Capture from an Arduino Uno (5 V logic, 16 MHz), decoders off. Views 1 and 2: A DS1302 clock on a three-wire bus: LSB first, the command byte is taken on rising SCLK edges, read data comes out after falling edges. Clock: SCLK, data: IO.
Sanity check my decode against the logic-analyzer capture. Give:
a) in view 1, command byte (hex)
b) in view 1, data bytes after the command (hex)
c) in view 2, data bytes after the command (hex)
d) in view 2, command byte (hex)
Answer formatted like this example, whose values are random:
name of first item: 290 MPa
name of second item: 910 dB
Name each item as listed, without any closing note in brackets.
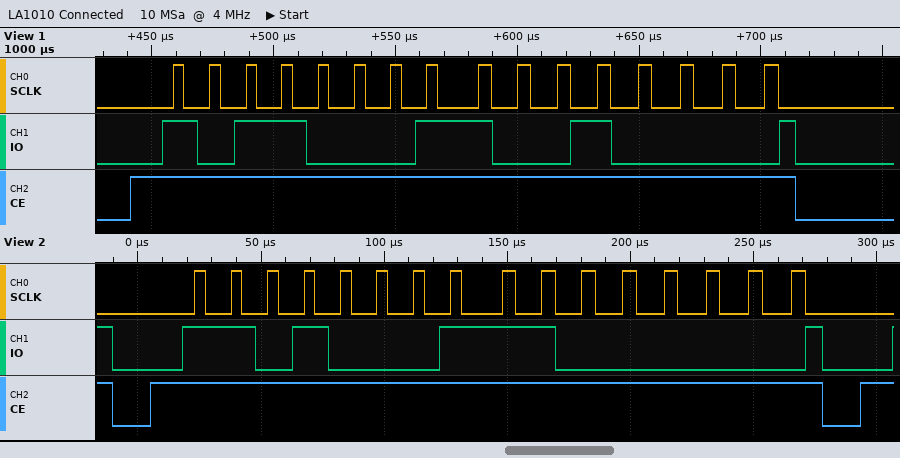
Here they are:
in view 1, command byte: 0x8D
in view 1, data bytes after the command: 09
in view 2, data bytes after the command: 03
in view 2, command byte: 0x8B
